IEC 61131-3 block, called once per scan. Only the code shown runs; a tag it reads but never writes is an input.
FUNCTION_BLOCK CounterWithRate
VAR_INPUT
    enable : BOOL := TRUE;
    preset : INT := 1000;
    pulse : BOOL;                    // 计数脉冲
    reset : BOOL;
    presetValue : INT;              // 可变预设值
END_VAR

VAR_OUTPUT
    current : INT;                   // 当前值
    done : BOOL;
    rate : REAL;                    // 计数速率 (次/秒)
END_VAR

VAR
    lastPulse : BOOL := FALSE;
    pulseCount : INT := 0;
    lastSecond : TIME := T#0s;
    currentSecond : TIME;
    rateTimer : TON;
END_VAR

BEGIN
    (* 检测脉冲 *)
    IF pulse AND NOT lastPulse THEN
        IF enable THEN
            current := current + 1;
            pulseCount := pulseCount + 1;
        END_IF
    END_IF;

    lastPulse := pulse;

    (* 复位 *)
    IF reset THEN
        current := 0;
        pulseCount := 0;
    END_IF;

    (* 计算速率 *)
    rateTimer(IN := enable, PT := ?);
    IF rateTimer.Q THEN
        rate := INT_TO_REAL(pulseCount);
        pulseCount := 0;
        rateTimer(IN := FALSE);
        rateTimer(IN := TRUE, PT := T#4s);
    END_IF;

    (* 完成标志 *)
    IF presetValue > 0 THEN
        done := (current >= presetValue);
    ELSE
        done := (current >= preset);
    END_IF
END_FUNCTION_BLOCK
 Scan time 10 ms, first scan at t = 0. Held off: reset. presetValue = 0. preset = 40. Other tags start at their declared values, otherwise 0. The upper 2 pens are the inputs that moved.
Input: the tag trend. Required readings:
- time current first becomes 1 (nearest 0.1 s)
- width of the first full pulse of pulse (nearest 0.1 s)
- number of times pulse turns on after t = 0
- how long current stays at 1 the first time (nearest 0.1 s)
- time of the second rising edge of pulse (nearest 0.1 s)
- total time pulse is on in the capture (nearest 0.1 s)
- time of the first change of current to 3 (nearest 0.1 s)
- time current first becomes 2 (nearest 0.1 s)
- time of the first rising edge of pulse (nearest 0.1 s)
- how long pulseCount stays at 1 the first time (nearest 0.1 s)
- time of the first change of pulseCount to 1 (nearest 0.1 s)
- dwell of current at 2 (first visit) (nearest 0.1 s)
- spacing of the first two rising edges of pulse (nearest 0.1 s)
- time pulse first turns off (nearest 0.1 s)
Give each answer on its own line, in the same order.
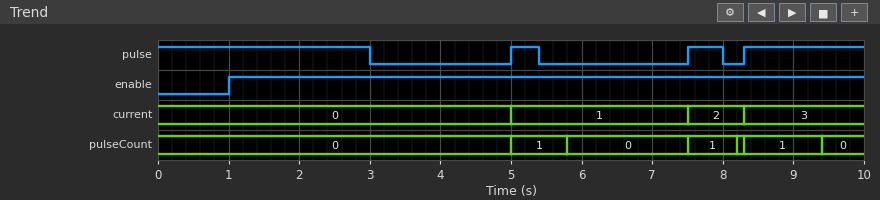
5.0 s
0.4 s
3
2.5 s
7.5 s
5.6 s
8.3 s
7.5 s
5.0 s
0.8 s
5.0 s
0.8 s
2.5 s
3.0 s
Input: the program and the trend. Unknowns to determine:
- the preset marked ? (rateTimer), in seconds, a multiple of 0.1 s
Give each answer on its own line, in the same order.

1.2 s
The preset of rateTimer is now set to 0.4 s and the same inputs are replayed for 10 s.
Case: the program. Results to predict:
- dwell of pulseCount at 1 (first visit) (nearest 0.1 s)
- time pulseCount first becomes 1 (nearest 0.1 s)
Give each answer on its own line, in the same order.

0.3 s
7.5 s
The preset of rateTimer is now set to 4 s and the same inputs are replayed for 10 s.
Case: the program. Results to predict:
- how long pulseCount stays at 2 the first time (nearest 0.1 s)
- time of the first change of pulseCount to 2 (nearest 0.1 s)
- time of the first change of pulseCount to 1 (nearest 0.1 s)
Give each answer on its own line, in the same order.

0.7 s
8.3 s
7.5 s
